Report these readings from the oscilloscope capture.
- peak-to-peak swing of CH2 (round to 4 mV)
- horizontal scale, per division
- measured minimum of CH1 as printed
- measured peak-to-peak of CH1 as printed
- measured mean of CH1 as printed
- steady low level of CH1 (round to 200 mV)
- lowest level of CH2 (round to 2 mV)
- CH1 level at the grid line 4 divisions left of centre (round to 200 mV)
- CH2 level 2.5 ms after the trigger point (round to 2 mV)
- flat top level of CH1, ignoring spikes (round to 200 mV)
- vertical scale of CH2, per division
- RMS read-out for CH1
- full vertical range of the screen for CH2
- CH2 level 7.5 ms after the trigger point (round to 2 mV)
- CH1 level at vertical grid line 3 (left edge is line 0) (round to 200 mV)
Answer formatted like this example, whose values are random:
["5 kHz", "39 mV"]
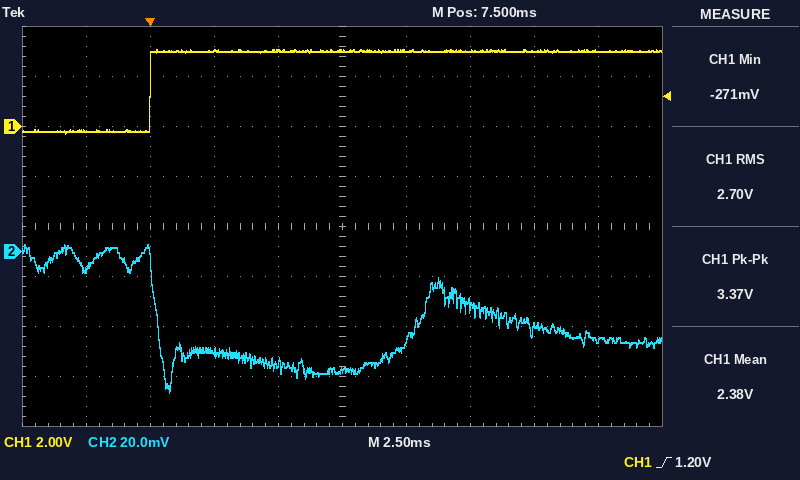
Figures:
["60 mV", "2.5 ms", "-271 mV", "3.37 V", "2.38 V", "-200 mV", "-56 mV", "-200 mV", "-40 mV", "3.0 V", "20 mV", "2.70 V", "160 mV", "-48 mV", "3.0 V"]
